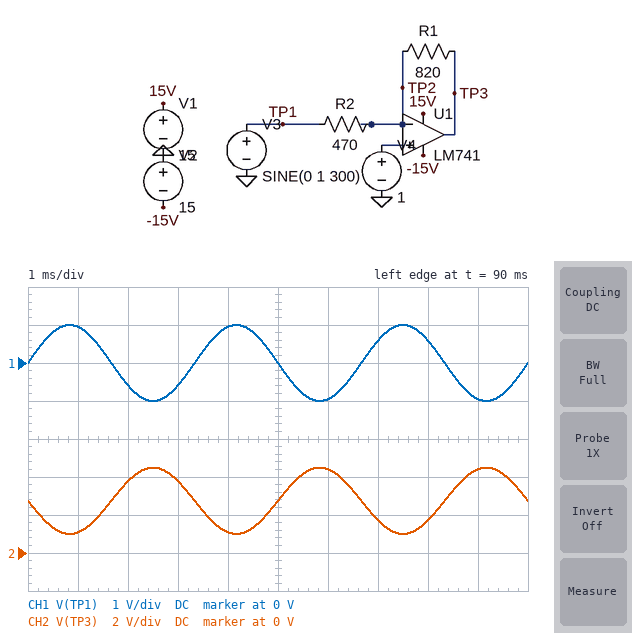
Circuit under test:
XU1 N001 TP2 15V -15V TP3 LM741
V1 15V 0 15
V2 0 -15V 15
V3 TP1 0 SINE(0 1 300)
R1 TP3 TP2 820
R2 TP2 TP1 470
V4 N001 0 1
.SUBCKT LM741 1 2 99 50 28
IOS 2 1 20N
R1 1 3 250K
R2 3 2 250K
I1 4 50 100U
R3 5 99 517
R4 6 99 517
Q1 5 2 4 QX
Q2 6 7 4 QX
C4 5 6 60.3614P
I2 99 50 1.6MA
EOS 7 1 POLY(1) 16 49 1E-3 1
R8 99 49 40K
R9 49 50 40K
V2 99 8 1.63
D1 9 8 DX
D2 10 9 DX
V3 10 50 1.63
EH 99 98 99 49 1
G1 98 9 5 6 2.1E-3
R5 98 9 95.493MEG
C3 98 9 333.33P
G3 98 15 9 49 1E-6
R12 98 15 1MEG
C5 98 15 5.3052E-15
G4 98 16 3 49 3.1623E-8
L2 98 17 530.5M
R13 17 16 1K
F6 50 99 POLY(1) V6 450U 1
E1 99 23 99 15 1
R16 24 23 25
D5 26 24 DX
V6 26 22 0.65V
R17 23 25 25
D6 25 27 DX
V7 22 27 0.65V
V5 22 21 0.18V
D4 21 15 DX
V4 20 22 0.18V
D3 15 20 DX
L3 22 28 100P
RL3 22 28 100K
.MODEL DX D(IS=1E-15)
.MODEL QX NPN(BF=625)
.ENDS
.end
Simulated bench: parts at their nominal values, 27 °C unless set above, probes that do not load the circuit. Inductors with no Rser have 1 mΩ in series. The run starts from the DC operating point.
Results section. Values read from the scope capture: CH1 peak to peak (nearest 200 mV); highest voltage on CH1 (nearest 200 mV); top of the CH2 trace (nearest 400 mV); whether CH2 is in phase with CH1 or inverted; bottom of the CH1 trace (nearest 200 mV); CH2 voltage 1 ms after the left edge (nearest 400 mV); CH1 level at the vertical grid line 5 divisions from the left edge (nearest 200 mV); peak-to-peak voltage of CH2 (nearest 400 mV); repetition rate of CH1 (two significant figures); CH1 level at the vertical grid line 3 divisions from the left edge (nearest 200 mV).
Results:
2.0 V
1.0 V
4.4 V
inverted
-1.0 V
1.2 V
0 V
3.6 V
300 Hz
-600 mV
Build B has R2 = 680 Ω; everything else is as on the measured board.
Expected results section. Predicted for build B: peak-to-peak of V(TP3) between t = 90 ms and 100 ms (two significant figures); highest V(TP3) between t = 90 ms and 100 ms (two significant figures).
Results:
2.4 V
3.4 V
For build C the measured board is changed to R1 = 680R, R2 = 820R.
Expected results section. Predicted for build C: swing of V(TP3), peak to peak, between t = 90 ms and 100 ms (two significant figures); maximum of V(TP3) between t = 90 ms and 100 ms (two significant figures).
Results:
1.7 V
2.7 V
